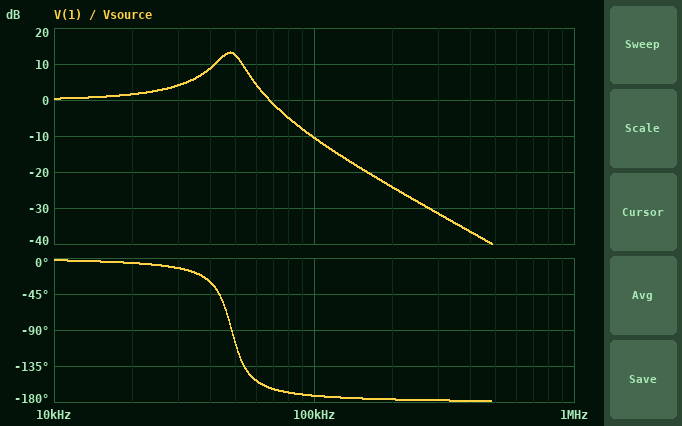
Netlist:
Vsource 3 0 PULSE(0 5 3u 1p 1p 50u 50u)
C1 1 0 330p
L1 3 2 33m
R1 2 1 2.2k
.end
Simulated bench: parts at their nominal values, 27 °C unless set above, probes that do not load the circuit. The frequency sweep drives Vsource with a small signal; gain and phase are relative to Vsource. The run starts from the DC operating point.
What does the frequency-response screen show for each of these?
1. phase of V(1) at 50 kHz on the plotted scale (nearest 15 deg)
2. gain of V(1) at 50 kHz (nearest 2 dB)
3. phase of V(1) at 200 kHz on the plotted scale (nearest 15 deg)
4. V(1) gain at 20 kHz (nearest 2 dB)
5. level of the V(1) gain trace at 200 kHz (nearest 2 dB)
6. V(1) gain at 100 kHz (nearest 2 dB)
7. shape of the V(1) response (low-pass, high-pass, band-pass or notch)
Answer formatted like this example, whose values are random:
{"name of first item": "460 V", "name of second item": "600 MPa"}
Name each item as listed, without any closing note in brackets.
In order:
{"phase of V(1) at 50 kHz on the plotted scale": "-105 deg", "gain of V(1) at 50 kHz": "12 dB", "phase of V(1) at 200 kHz on the plotted scale": "-180 deg", "V(1) gain at 20 kHz": "2 dB", "level of the V(1) gain trace at 200 kHz": "-24 dB", "V(1) gain at 100 kHz": "-10 dB", "shape of the V(1) response": "low-pass"}
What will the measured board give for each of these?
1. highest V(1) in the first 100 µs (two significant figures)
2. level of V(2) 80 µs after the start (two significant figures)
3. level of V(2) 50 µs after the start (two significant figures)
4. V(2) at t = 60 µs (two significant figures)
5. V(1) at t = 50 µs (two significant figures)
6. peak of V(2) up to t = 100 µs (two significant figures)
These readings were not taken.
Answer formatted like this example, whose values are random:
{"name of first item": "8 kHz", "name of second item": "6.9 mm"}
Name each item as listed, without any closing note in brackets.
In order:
{"highest V(1) in the first 100 µs": "8.5 V", "level of V(2) 80 µs after the start": "5.1 V", "level of V(2) 50 µs after the start": "5.1 V", "V(2) at t = 60 µs": "5.0 V", "V(1) at t = 50 µs": "4.9 V", "peak of V(2) up to t = 100 µs": "8.6 V"}
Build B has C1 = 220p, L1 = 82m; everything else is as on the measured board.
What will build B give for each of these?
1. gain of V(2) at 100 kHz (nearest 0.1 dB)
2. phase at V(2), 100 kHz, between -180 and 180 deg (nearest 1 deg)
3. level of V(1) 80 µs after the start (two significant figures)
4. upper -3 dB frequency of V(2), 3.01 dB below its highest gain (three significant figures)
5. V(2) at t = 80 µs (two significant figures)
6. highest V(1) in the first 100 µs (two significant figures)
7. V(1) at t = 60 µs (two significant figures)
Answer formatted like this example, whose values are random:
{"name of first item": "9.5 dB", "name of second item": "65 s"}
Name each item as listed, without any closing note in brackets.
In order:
{"gain of V(2) at 100 kHz": "-15.4 dB", "phase at V(2), 100 kHz, between -180 and 180 deg": "-160 deg", "level of V(1) 80 µs after the start": "3.8 V", "upper -3 dB frequency of V(2), 3.01 dB below its highest gain": "39.4 kHz", "V(2) at t = 80 µs": "3.6 V", "highest V(1) in the first 100 µs": "9.2 V", "V(1) at t = 60 µs": "3.3 V"}
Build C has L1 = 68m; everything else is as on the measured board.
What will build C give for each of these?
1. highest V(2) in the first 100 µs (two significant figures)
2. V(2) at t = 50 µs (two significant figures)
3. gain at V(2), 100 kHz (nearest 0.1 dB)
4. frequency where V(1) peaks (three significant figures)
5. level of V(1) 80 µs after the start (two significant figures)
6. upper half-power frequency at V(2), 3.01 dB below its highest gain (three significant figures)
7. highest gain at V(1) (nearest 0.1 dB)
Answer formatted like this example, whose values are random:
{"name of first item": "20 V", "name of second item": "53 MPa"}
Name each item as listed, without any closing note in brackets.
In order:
{"highest V(2) in the first 100 µs": "9.0 V", "V(2) at t = 50 µs": "7.0 V", "gain at V(2), 100 kHz": "-17.1 dB", "frequency where V(1) peaks": "33.4 kHz", "level of V(1) 80 µs after the start": "6.3 V", "upper half-power frequency at V(2), 3.01 dB below its highest gain": "35.9 kHz", "highest gain at V(1)": "16.3 dB"}
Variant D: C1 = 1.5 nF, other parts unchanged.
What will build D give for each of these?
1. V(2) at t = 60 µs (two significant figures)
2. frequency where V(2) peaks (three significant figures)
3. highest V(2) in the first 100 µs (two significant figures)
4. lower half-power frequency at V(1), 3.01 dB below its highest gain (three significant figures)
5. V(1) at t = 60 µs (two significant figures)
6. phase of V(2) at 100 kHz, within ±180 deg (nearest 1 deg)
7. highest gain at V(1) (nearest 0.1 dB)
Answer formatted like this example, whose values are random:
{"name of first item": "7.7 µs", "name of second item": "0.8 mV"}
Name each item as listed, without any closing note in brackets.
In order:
{"V(2) at t = 60 µs": "5.2 V", "frequency where V(2) peaks": "21.6 kHz", "highest V(2) in the first 100 µs": "7.6 V", "lower half-power frequency at V(1), 3.01 dB below its highest gain": "14.9 kHz", "V(1) at t = 60 µs": "4.8 V", "phase of V(2) at 100 kHz, within ±180 deg": "-109 deg", "highest gain at V(1)": "6.8 dB"}
